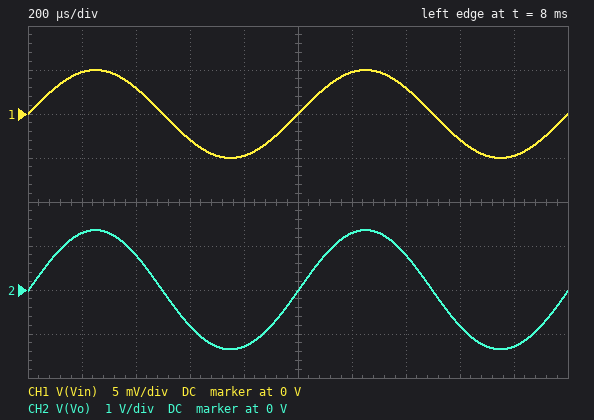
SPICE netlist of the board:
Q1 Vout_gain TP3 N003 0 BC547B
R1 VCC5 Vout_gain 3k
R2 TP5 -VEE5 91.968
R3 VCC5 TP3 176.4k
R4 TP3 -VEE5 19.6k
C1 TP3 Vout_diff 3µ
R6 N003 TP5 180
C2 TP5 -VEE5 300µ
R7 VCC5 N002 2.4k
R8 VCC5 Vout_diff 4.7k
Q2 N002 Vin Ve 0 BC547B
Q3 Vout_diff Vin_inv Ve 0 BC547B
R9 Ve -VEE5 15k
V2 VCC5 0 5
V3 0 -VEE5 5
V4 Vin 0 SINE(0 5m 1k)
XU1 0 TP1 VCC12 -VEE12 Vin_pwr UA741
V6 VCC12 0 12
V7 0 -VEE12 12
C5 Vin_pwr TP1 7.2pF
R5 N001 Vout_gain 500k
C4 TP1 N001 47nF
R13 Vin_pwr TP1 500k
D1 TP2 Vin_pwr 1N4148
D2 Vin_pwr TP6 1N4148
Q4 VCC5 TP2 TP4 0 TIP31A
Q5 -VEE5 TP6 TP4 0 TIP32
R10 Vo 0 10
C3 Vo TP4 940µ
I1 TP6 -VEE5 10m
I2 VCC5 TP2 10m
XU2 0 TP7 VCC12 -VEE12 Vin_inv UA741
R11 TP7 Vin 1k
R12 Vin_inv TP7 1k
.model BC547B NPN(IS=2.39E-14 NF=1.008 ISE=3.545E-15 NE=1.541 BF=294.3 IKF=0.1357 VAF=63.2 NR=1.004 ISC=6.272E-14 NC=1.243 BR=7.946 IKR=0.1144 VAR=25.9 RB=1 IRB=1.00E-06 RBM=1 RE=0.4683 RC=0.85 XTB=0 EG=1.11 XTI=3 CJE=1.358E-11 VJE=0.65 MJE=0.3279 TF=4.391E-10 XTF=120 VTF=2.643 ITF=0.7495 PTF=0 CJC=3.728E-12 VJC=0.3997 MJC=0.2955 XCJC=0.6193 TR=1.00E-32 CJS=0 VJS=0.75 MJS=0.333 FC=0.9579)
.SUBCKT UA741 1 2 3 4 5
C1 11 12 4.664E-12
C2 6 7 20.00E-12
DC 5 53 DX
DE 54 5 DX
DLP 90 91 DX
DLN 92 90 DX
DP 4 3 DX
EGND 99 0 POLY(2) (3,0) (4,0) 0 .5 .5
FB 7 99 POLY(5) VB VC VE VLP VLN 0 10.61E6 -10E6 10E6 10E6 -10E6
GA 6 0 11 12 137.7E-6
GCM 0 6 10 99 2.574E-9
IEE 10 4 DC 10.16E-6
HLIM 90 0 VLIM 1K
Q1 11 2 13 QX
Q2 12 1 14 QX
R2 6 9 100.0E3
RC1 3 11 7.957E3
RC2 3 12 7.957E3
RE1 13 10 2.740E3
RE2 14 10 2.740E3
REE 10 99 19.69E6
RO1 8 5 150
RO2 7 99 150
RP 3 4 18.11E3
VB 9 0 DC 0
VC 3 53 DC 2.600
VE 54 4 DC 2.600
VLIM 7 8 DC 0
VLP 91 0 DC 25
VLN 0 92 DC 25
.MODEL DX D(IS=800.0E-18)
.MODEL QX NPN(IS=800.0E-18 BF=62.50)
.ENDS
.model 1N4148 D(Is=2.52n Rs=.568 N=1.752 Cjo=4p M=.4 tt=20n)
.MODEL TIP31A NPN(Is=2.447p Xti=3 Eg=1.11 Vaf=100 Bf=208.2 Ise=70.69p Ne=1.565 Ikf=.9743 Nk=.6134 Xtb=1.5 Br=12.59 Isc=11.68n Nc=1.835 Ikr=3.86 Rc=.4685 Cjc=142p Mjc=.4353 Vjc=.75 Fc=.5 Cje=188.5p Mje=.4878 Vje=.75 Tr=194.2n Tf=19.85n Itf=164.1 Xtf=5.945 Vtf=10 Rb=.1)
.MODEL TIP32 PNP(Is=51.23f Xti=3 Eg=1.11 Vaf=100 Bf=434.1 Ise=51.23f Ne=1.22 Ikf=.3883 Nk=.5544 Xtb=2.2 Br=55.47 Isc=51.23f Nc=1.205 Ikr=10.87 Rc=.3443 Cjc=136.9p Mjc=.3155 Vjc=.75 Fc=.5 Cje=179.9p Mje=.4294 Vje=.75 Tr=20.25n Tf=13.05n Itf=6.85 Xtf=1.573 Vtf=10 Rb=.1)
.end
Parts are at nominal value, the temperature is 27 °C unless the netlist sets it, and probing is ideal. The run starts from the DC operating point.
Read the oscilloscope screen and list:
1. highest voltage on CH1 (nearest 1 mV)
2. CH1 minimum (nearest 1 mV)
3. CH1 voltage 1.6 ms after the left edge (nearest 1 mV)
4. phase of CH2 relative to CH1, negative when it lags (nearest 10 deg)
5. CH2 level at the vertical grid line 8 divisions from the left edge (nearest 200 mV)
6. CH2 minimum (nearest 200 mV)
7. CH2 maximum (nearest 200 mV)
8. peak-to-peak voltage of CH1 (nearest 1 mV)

5 mV
-5 mV
-3 mV
0 deg
-800 mV
-1.4 V
1.4 V
10 mV
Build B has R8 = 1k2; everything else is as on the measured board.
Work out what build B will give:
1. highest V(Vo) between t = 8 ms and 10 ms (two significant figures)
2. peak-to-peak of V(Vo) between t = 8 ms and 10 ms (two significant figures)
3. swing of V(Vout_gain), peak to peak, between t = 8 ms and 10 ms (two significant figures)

430 mV
860 mV
880 mV
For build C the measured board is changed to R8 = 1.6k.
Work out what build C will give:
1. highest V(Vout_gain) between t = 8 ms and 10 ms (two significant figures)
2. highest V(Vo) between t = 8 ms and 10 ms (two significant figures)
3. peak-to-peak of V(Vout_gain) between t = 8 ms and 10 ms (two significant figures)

2.3 V
560 mV
1.1 V
